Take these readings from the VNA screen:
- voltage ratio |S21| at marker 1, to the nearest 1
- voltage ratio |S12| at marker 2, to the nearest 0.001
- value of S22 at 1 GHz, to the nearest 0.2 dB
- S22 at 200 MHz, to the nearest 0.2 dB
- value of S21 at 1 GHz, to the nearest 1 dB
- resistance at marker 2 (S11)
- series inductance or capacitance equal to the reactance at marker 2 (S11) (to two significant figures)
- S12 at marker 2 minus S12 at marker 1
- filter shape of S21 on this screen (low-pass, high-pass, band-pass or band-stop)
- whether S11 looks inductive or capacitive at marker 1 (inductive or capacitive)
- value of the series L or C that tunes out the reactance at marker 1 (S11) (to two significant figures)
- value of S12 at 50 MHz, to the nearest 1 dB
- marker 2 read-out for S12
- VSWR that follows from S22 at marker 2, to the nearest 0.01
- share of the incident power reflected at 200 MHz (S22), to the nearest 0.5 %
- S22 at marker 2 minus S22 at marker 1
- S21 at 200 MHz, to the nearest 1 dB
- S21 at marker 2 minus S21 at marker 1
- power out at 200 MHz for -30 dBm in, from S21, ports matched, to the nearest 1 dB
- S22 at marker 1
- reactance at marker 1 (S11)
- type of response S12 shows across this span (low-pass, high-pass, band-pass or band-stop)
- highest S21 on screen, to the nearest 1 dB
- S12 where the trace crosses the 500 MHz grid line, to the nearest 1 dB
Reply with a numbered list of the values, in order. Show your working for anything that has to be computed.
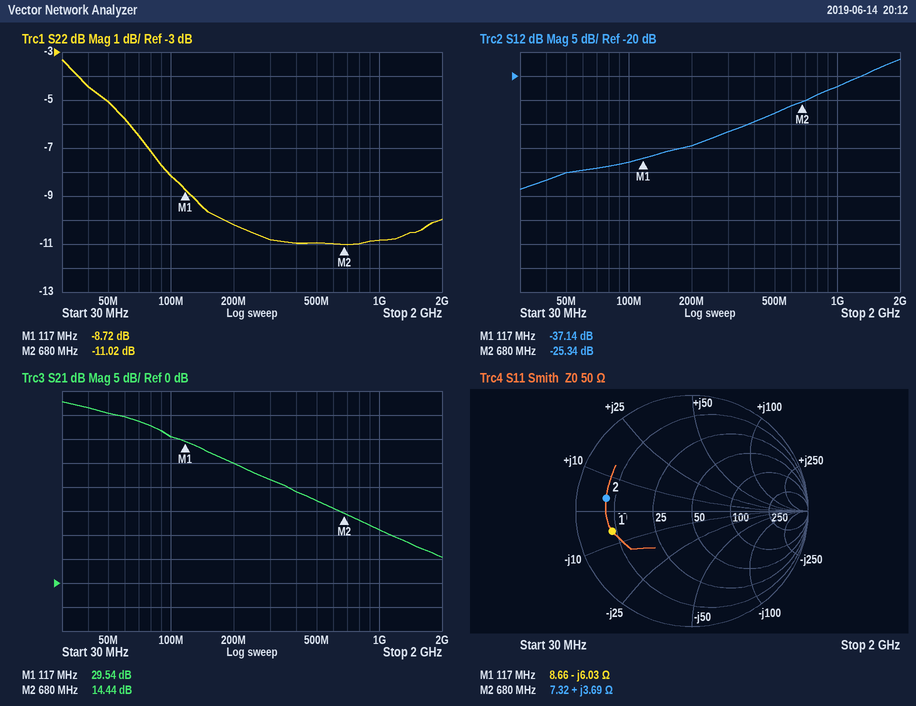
1. 10^(29.54/20) ≈ 30
2. 10^(-25.34/20) ≈ 0.054
3. -10.8 dB
4. -10.2 dB
5. 11 dB
6. 7.32 Ω
7. L = 3.69 Ω/(2π × 680 MHz) ≈ 864 pH, so 860 pH to two significant figures
8. -25.34 − (-37.14) = 11.80 dB
9. low-pass
10. capacitive
11. L = 6.03 Ω/(2π × 117 MHz) ≈ 8.2 nH
12. -40 dB
13. -25.34 dB
14. (1 + 0.2812)/(1 − 0.2812) ≈ 1.78
15. 10^(-10.2/10) ≈ 9.5 %
16. -11.02 − (-8.72) = -2.30 dB
17. 25 dB
18. 14.44 − (29.54) = -15.10 dB
19. -30 dBm + (25 dB) = -5 dBm
20. -8.72 dB
21. -6.03 Ω
22. high-pass
23. 38 dB
24. -28 dB
